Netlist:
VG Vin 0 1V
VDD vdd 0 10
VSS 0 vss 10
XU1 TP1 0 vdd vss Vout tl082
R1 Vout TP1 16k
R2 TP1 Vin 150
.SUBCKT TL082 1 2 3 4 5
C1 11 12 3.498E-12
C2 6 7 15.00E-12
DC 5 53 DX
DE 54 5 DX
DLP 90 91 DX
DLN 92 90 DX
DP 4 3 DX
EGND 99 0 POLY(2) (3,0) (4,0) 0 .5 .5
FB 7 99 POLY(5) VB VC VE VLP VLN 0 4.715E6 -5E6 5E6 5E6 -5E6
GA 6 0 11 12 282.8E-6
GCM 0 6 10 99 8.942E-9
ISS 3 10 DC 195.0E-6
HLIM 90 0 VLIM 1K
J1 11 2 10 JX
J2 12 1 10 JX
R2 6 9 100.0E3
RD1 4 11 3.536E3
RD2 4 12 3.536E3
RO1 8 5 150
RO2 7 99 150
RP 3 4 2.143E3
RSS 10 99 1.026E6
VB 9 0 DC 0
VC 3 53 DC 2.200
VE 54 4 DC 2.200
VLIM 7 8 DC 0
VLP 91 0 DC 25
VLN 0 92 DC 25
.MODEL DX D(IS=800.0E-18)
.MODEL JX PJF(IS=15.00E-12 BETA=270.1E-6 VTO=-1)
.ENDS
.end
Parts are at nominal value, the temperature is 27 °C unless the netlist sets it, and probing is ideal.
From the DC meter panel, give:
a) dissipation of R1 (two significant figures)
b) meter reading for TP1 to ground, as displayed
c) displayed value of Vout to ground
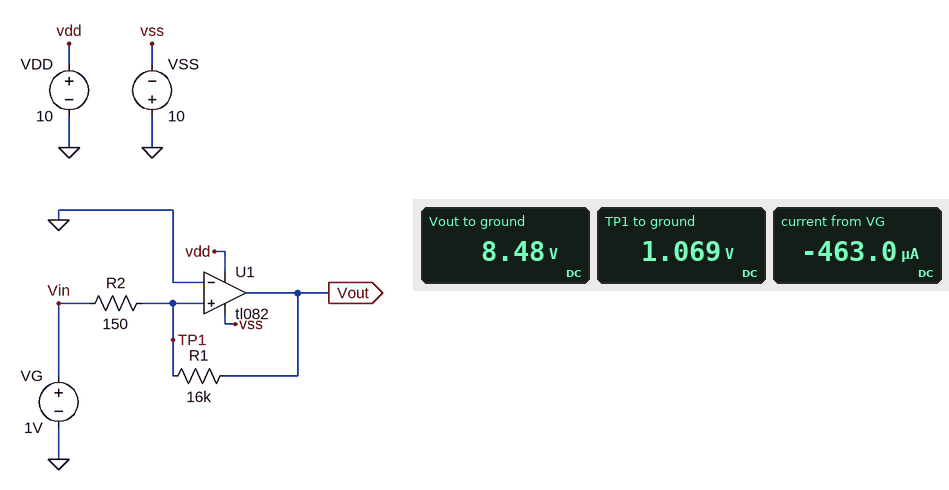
3.4 mW
1.069 V
8.48 V
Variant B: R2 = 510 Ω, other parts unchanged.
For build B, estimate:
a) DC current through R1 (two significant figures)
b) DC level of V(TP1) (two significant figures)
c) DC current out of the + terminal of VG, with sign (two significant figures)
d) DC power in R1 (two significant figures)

450 µA
1.2 V
-450 µA
3.3 mW
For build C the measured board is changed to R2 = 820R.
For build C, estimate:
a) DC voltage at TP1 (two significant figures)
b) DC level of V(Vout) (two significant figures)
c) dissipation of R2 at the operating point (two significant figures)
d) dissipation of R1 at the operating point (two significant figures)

1.4 V
8.5 V
160 µW
3.2 mW
